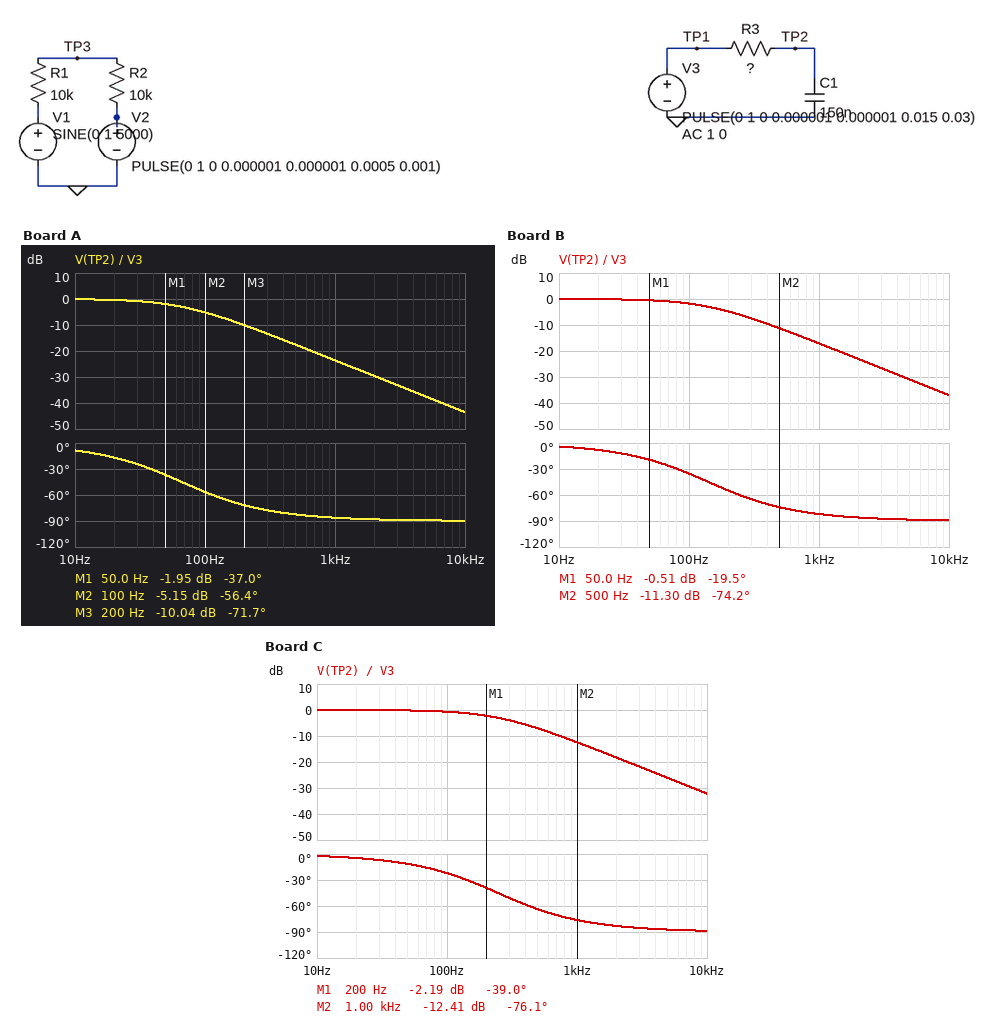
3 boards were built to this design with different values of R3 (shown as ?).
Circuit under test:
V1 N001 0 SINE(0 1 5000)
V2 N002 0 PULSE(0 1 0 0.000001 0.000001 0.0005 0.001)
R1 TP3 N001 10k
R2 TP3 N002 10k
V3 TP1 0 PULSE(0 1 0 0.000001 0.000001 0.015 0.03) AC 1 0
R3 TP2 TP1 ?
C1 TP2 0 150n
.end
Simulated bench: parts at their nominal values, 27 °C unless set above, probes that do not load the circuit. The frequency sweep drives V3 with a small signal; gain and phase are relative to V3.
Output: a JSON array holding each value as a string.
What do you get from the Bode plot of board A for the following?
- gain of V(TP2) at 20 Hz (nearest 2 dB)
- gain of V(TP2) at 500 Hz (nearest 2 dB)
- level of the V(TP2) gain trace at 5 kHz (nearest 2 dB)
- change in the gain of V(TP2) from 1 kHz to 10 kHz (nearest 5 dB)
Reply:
["0 dB", "-18 dB", "-38 dB", "-20 dB"]
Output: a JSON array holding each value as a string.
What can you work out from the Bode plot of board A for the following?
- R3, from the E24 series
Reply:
["16 kΩ"]
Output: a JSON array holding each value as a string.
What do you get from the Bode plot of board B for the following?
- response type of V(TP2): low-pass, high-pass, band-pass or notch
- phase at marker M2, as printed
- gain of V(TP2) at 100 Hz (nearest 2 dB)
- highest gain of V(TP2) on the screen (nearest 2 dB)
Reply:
["low-pass", "-74.2 deg", "-2 dB", "0 dB"]
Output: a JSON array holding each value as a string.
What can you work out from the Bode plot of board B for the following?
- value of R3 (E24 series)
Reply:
["7.5 kΩ"]
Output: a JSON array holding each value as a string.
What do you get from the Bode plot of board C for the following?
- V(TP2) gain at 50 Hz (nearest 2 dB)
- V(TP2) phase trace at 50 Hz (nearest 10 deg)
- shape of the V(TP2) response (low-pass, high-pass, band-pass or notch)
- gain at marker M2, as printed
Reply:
["0 dB", "-10 deg", "low-pass", "-12.41 dB"]
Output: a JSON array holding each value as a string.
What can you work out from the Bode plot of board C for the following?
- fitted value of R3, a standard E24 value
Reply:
["4.3 kΩ"]
